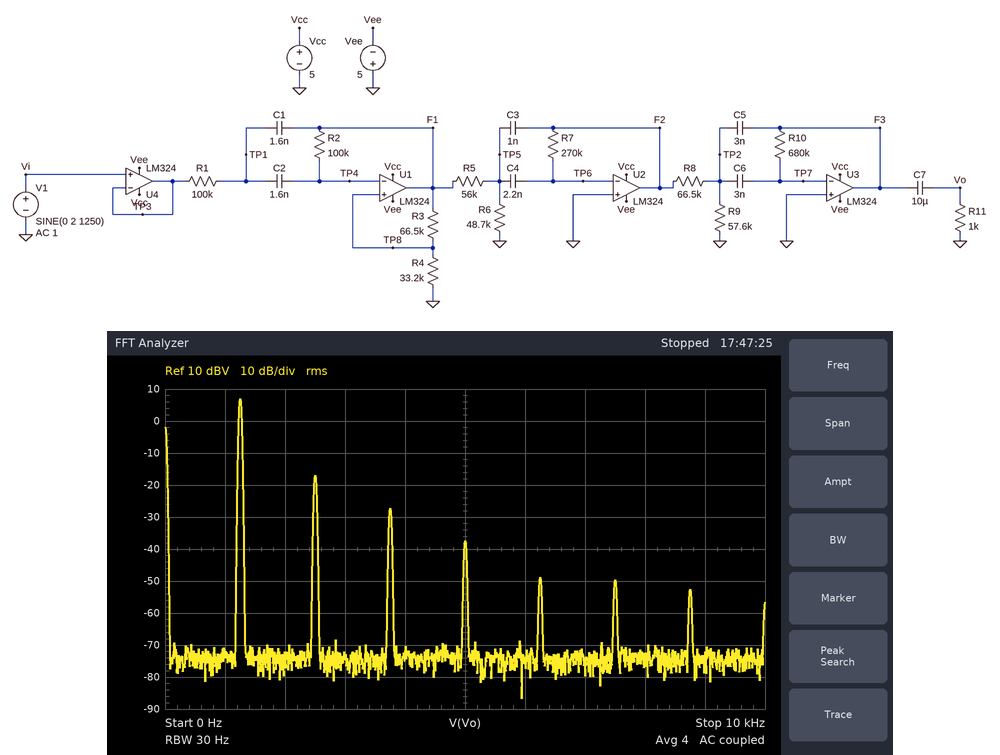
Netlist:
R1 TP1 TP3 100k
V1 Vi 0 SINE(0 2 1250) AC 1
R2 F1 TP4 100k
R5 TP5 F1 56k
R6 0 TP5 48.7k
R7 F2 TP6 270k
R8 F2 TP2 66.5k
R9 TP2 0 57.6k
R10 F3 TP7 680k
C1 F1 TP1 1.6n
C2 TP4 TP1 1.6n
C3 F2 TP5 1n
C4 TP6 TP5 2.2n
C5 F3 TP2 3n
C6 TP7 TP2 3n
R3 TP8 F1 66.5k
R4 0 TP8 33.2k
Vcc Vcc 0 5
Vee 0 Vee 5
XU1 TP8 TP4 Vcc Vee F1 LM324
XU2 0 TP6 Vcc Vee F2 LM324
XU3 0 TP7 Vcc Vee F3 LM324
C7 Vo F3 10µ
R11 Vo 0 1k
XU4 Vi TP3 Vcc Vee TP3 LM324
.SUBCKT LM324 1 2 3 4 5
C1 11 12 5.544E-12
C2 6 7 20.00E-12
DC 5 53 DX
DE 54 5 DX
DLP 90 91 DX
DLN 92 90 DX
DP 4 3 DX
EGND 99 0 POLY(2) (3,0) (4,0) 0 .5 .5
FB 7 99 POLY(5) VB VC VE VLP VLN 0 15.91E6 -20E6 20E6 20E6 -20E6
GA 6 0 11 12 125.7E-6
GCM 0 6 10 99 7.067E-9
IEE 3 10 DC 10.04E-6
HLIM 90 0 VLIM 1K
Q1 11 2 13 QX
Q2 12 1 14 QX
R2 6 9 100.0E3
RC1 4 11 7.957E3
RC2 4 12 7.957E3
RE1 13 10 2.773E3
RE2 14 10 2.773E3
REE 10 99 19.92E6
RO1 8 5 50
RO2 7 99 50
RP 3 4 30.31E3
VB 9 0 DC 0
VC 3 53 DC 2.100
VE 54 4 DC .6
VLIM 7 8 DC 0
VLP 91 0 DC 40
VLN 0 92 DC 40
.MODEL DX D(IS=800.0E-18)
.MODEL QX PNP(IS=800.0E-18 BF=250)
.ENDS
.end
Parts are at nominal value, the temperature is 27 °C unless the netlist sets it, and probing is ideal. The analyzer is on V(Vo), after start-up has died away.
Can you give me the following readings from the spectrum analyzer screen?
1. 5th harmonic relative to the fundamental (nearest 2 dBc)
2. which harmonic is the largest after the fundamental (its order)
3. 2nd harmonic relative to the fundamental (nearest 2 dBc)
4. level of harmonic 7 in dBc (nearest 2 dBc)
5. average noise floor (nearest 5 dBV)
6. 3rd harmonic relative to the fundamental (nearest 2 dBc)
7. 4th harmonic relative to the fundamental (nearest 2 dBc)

-56 dBc
2
-24 dBc
-60 dBc
-75 dBV
-34 dBc
-44 dBc
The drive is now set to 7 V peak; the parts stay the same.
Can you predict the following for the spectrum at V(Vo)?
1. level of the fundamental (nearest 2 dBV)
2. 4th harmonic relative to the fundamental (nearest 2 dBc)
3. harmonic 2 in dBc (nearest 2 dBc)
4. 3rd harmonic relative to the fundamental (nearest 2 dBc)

6 dBV
-42 dBc
-16 dBc
-24 dBc
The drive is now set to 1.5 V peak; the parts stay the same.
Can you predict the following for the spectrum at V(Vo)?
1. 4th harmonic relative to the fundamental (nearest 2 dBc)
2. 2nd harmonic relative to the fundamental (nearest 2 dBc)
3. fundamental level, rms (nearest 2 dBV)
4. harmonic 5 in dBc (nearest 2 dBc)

-46 dBc
-30 dBc
6 dBV
-52 dBc
